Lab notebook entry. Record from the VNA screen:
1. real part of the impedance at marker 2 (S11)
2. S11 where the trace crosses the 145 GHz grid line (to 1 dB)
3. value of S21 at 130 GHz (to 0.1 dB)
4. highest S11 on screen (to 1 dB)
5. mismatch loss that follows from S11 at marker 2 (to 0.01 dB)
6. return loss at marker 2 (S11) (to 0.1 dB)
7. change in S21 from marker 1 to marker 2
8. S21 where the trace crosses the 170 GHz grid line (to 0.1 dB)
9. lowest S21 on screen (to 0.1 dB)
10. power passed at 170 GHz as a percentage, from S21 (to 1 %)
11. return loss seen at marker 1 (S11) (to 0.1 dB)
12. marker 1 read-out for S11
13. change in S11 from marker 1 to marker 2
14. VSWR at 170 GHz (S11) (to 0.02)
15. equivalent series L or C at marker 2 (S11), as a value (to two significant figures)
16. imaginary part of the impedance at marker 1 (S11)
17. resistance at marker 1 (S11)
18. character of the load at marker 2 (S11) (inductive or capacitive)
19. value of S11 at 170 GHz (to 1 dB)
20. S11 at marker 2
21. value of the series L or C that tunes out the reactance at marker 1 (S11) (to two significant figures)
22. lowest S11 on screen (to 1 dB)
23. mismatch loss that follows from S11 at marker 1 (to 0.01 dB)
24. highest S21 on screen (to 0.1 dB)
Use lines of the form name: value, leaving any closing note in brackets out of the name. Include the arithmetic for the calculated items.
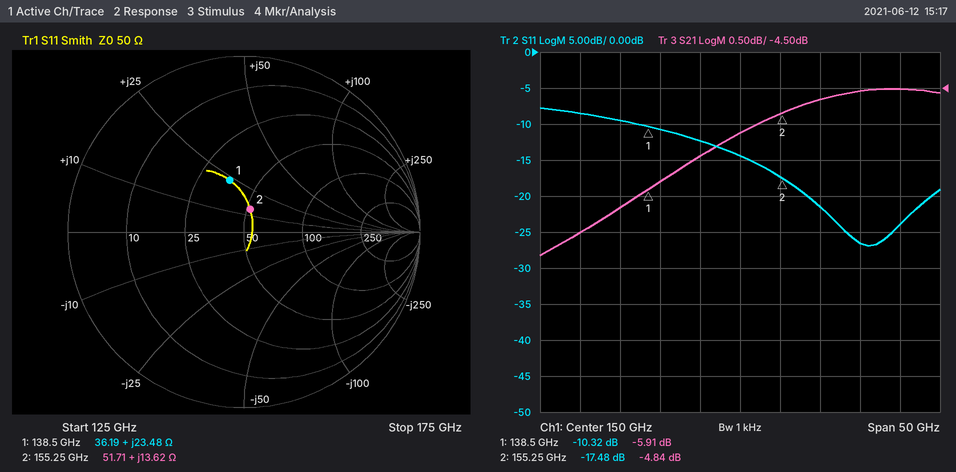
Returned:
real part of the impedance at marker 2: 51.71 Ω
S11 where the trace crosses the 145 GHz grid line: -12 dB
value of S21 at 130 GHz: -6.5 dB
highest S11 on screen: -8 dB
mismatch loss that follows from S11 at marker 2: −10 log10(1 − 10^(-17.48/10)) ≈ 0.08 dB
return loss at marker 2 (S11): 17.5 dB
change in S21 from marker 1 to marker 2: -4.84 − (-5.91) = 1.07 dB
S21 where the trace crosses the 170 GHz grid line: -4.5 dB
lowest S21 on screen: -6.8 dB
power passed at 170 GHz as a percentage, from S21: 10^(-4.5/10) ≈ 35 %
return loss seen at marker 1 (S11): 10.3 dB
marker 1 read-out for S11: -10.32 dB
change in S11 from marker 1 to marker 2: -17.48 − (-10.32) = -7.16 dB
VSWR at 170 GHz (S11): |Γ| = 10^(-24/20) = 0.0631; VSWR = (1 + 0.0631)/(1 − 0.0631) ≈ 1.13, so 1.14 to the nearest 0.02
equivalent series L or C at marker 2 (S11), as a value: L = 13.62 Ω/(2π × 155.25 GHz) ≈ 14 pH
imaginary part of the impedance at marker 1: +23.48 Ω
resistance at marker 1: 36.19 Ω
character of the load at marker 2 (S11): inductive
value of S11 at 170 GHz: -24 dB
S11 at marker 2: -17.48 dB
value of the series L or C that tunes out the reactance at marker 1 (S11): C = 1/(2π × 138.5 GHz × 23.48 Ω) ≈ 49 fF
lowest S11 on screen: -27 dB
mismatch loss that follows from S11 at marker 1: −10 log10(1 − 10^(-10.32/10)) ≈ 0.42 dB
highest S21 on screen: -4.5 dB
